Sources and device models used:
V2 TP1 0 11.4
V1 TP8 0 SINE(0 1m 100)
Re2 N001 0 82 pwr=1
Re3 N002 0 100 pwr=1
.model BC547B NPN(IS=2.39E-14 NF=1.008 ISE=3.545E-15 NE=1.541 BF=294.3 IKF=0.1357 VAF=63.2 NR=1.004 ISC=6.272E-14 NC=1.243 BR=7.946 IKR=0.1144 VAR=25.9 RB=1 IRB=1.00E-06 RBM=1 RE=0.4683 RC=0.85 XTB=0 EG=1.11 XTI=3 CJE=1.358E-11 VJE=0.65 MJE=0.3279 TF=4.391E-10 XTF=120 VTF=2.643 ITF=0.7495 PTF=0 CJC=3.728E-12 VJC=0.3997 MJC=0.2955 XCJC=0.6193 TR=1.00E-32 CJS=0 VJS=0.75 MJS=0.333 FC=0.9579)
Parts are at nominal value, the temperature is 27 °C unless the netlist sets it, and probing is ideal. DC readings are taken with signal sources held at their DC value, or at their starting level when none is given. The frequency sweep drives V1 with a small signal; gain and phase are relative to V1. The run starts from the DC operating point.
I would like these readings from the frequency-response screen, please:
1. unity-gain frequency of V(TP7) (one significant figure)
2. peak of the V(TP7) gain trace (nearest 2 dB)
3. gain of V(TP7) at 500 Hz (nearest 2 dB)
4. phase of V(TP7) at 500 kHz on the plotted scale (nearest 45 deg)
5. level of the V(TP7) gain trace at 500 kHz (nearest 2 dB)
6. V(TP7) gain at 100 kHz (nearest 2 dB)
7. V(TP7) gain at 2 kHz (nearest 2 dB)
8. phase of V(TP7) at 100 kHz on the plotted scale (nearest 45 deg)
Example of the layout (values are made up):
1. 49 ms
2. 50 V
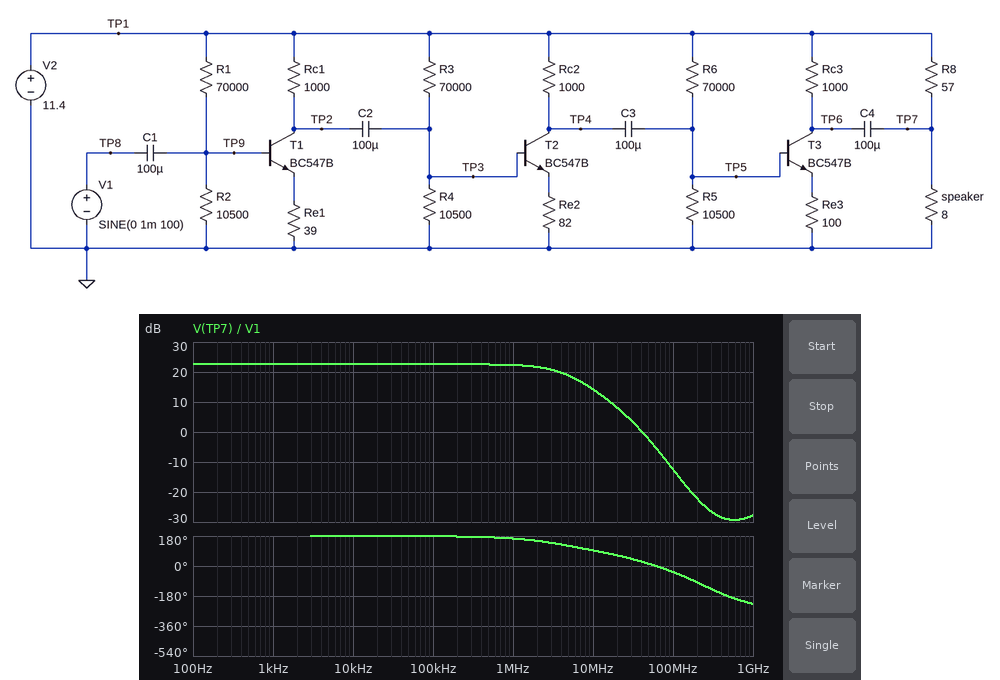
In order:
1. 40 MHz
2. 22 dB
3. 22 dB
4. 180 deg
5. 22 dB
6. 22 dB
7. 22 dB
8. 180 deg
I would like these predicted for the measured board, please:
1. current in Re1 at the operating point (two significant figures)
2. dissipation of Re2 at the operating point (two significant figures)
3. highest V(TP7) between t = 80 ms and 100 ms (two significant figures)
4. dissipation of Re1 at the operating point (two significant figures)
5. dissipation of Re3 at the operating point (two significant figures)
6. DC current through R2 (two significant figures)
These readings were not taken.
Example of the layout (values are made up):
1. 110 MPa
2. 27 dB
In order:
1. 11 mA
2. 4.0 mW
3. 1.4 V
4. 4.4 mW
5. 3.7 mW
6. 110 µA
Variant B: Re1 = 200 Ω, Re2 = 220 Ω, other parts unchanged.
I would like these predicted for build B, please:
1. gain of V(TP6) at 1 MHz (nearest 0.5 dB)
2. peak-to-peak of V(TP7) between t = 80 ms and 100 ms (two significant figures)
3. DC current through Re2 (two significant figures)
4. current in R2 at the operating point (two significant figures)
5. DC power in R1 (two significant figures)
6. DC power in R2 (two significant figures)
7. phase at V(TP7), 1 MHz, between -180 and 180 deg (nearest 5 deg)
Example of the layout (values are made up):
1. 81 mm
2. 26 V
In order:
1. 0.5 dB
2. 2.1 mV
3. 3.3 mA
4. 130 µA
5. 1.4 mW
6. 180 µW
7. 170 deg
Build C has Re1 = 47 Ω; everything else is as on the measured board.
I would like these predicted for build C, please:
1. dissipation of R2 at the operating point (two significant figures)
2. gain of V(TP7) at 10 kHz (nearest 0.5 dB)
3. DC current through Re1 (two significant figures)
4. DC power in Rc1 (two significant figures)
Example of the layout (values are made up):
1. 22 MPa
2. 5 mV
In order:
1. 130 µW
2. 21.0 dB
3. 9.7 mA
4. 93 mW
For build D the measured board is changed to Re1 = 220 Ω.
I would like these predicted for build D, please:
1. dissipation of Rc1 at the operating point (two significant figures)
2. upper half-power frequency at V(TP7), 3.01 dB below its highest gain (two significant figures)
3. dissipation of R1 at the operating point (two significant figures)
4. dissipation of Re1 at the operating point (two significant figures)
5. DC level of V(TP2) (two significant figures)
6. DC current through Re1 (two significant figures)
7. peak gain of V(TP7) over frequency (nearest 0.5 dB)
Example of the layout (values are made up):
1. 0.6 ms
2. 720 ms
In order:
1. 11 mW
2. 4.5 MHz
3. 1.4 mW
4. 2.4 mW
5. 8.1 V
6. 3.3 mA
7. 8.0 dB
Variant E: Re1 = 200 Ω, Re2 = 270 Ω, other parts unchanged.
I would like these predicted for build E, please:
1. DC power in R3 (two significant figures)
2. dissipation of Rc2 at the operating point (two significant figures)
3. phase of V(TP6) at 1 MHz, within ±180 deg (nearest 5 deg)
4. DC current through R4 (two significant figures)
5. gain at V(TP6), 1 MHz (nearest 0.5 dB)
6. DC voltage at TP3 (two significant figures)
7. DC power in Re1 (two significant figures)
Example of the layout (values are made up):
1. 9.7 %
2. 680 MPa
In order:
1. 1.4 mW
2. 7.5 mW
3. 170 deg
4. 130 µA
5. -1.0 dB
6. 1.4 V
7. 2.5 mW
